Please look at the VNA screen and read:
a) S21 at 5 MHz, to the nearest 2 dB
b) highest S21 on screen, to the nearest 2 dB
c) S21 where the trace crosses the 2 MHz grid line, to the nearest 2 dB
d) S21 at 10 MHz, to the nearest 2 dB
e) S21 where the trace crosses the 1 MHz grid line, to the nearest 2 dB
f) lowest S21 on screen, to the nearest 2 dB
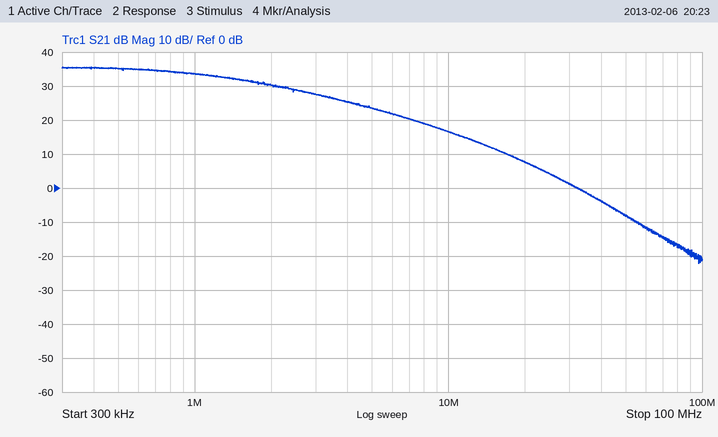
24 dB
36 dB
30 dB
16 dB
34 dB
-22 dB
